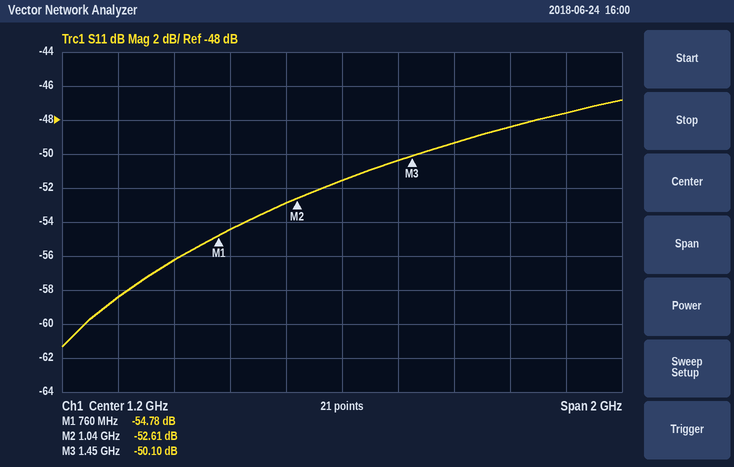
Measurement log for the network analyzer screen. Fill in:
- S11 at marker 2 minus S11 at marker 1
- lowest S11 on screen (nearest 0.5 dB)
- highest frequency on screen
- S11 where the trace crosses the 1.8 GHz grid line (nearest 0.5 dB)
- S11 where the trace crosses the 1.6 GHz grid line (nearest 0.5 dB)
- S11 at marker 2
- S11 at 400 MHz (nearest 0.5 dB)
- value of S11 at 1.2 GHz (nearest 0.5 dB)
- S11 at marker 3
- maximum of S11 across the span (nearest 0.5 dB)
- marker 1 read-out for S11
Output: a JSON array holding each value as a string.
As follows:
["2.17 dB", "-61.5 dB", "2.2 GHz", "-48.5 dB", "-49.5 dB", "-52.61 dB", "-58.5 dB", "-51.5 dB", "-50.10 dB", "-47.0 dB", "-54.78 dB"]
